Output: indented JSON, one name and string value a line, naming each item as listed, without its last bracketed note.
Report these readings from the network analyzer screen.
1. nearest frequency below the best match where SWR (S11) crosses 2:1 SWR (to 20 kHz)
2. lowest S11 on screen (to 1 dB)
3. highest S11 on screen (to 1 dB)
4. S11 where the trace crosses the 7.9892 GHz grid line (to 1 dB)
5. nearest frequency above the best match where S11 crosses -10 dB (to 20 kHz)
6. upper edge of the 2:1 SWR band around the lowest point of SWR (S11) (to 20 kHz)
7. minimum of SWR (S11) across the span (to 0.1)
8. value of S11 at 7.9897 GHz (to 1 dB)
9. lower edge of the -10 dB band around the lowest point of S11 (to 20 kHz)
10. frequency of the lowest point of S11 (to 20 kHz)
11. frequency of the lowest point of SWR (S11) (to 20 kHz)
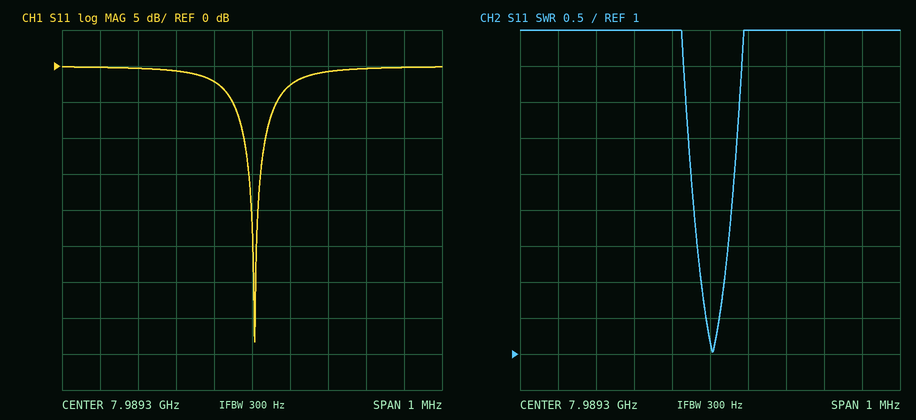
{
  "nearest frequency below the best match where SWR (S11) crosses 2:1 SWR": "7.98928 GHz",
  "lowest S11 on screen": "-38 dB",
  "highest S11 on screen": "0 dB",
  "S11 where the trace crosses the 7.9892 GHz grid line": "-2 dB",
  "nearest frequency above the best match where S11 crosses -10 dB": "7.98934 GHz",
  "upper edge of the 2:1 SWR band around the lowest point of SWR (S11)": "7.98934 GHz",
  "minimum of SWR (S11) across the span": "1.0",
  "value of S11 at 7.9897 GHz": "0 dB",
  "lower edge of the -10 dB band around the lowest point of S11": "7.98928 GHz",
  "frequency of the lowest point of S11": "7.98930 GHz",
  "frequency of the lowest point of SWR (S11)": "7.98930 GHz"
}
